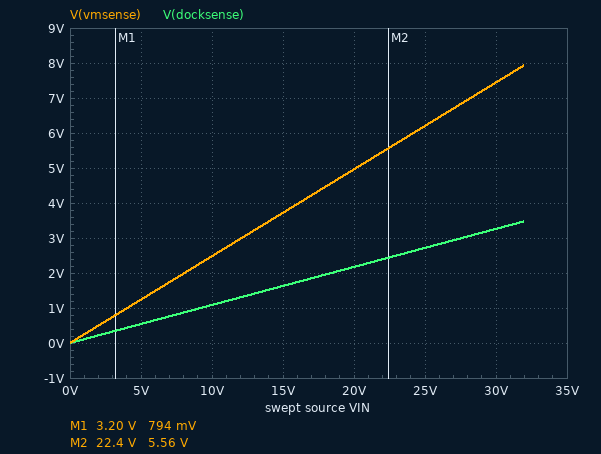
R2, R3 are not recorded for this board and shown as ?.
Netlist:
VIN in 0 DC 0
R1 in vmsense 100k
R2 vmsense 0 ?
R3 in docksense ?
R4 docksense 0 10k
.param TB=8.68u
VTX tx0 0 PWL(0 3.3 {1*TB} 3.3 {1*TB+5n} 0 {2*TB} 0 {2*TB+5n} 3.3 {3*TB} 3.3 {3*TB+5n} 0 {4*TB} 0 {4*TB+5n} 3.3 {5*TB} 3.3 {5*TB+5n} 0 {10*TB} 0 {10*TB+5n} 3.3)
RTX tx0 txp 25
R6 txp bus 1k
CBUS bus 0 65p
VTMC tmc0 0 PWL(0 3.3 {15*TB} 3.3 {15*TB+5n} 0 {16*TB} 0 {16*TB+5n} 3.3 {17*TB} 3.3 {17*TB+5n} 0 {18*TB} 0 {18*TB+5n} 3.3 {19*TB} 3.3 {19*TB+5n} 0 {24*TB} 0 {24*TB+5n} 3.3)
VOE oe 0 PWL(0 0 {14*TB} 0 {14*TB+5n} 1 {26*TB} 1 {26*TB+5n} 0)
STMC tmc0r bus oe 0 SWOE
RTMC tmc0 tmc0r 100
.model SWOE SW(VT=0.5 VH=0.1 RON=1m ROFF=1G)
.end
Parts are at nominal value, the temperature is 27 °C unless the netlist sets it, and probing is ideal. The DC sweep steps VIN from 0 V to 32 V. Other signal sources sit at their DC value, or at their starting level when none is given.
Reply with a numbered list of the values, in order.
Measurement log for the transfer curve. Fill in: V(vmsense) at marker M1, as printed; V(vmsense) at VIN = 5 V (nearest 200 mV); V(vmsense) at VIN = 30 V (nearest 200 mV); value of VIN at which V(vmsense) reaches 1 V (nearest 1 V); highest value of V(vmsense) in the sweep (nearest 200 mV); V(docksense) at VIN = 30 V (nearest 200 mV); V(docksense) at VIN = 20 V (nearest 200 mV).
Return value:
1. 794 mV
2. 1.2 V
3. 7.4 V
4. 4 V
5. 8.0 V
6. 3.2 V
7. 2.2 V
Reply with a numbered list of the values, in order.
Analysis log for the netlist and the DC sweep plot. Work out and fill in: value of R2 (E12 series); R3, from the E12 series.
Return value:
1. 33 kΩ
2. 82 kΩ
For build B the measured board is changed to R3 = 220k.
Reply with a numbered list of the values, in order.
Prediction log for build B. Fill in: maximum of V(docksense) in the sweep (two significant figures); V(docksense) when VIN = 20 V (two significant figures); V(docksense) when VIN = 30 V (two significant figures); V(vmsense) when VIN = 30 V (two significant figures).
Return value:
1. 1.4 V
2. 870 mV
3. 1.3 V
4. 7.4 V
